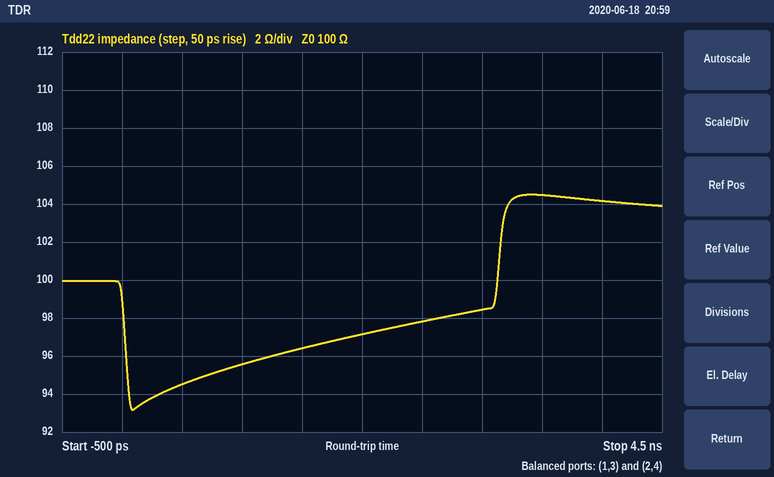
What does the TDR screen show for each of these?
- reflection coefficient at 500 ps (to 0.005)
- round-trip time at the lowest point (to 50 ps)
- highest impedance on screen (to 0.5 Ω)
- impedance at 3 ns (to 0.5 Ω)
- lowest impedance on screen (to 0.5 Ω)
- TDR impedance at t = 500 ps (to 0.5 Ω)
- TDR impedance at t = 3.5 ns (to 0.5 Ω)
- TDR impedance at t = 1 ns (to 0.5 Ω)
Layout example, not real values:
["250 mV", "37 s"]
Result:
["-0.030", "100 ps", "104.5 Ω", "98.5 Ω", "93.0 Ω", "94.5 Ω", "104.5 Ω", "95.5 Ω"]
